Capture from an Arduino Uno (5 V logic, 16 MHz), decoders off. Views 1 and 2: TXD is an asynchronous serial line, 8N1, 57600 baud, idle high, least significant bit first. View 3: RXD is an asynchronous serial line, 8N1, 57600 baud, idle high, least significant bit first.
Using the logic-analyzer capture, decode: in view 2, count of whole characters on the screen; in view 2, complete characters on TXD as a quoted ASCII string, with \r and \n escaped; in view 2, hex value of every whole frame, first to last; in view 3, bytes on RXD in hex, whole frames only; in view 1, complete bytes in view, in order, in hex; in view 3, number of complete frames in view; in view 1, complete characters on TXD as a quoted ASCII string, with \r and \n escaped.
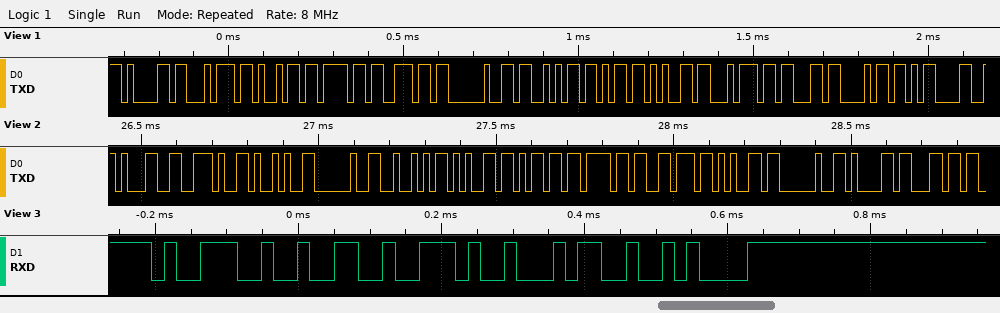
13
"1.) Remove al"
0x31 0x2E 0x29 0x20 0x52 0x65 0x6D 0x6F 0x76 0x65 0x20 0x61 0x6C
0x39 0x32 0x2E 0x34 0x0A
0x61 0x74 0x69 0x6F 0x6E 0x20 0x53 0x6B 0x65 0x74 0x63 0x68 0x0D
5
"ation Sketch\r"
